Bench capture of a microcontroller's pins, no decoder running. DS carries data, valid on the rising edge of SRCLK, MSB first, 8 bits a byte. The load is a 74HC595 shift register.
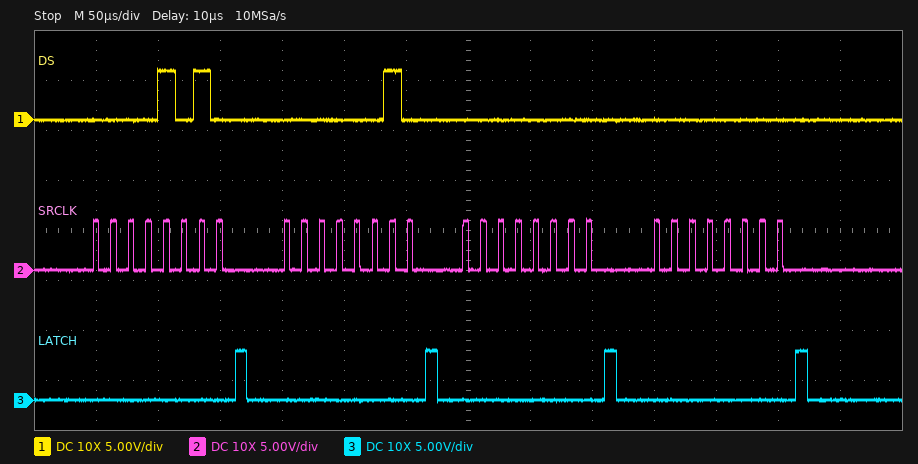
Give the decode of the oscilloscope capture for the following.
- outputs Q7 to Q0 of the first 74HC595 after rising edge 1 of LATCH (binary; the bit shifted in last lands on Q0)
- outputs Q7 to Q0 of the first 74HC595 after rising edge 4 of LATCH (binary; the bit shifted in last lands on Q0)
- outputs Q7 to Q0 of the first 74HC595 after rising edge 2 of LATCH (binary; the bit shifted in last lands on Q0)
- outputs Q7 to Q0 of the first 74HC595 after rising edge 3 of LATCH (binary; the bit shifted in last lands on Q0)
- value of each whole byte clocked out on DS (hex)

00001010
00000000
00000010
00000000
0A 02 00 00
